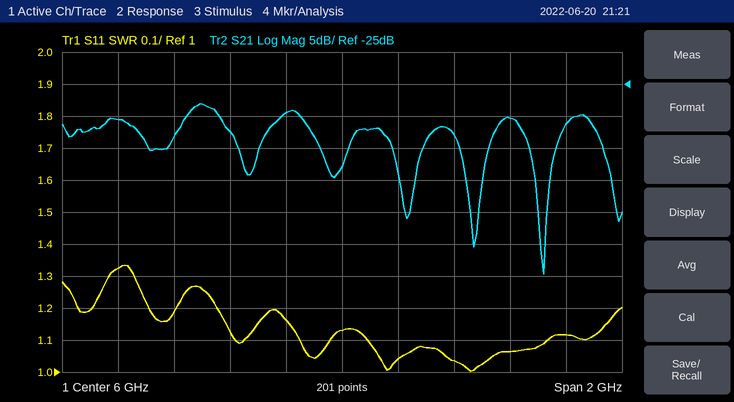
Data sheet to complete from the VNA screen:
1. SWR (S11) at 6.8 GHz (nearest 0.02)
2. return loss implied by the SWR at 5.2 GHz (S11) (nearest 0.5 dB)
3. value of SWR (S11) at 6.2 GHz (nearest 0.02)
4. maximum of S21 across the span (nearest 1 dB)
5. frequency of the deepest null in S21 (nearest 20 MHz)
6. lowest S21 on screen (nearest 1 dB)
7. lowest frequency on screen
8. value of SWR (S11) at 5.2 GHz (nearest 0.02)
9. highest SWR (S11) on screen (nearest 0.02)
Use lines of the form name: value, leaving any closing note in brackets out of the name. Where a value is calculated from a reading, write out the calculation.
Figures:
SWR (S11) at 6.8 GHz: 1.12
return loss implied by the SWR at 5.2 GHz (S11): −20 log10((1.32 − 1)/(1.32 + 1)) ≈ 17.2 dB, so 17.0 dB to the nearest 0.5 dB
value of SWR (S11) at 6.2 GHz: 1.04
maximum of S21 across the span: -28 dB
frequency of the deepest null in S21: 6.72 GHz
lowest S21 on screen: -55 dB
lowest frequency on screen: 5 GHz
value of SWR (S11) at 5.2 GHz: 1.32
highest SWR (S11) on screen: 1.34
